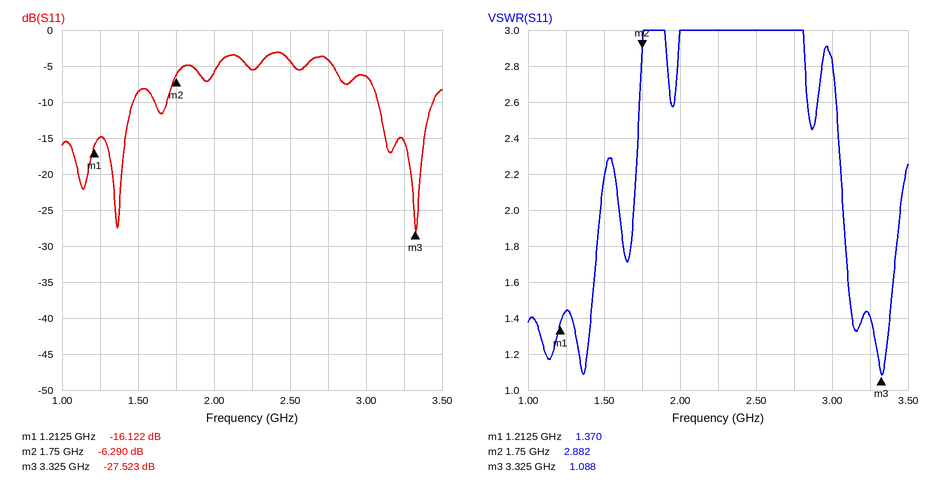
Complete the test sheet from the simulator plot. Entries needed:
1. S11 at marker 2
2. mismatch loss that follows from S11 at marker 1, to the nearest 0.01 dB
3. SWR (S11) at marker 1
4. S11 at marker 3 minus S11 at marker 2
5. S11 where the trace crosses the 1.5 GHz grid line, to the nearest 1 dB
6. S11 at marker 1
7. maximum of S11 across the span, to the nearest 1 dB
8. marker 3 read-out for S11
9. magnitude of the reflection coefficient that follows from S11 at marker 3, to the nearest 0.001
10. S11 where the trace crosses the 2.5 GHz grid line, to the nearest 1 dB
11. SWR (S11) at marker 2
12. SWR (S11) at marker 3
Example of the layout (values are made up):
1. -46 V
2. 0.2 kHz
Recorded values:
1. -6.290 dB
2. 0.11 dB
3. 1.370
4. -21.233 dB
5. -9 dB
6. -16.122 dB
7. -3 dB
8. -27.523 dB
9. 0.042
10. -4 dB
11. 2.882
12. 1.088
